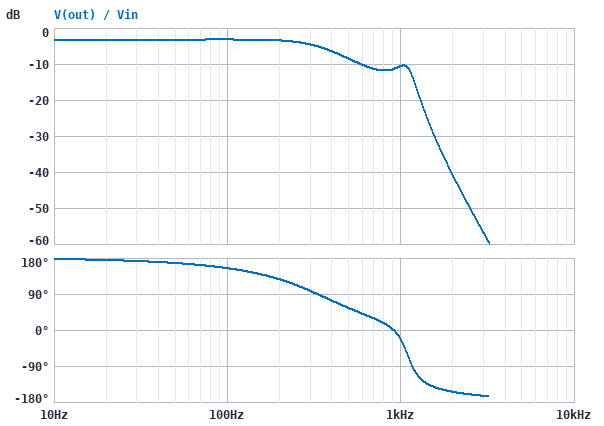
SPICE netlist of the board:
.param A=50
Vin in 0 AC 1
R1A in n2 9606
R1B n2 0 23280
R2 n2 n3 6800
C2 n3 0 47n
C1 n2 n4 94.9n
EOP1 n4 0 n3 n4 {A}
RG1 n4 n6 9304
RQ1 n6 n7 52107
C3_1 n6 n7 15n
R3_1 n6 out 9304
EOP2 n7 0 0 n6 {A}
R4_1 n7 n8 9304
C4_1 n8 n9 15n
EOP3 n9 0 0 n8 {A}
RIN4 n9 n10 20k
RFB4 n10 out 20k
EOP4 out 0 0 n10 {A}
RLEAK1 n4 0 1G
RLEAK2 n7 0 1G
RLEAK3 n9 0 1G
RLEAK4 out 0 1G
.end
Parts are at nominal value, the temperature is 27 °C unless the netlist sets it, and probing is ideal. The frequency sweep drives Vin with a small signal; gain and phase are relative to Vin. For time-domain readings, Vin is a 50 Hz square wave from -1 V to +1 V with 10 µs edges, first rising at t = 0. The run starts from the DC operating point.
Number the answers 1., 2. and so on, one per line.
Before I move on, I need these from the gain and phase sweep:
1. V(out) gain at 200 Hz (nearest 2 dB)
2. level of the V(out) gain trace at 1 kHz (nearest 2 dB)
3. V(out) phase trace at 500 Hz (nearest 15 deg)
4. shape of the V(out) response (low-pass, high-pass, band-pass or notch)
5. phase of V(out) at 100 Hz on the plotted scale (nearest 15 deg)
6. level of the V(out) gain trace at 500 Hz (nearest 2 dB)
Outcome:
1. -4 dB
2. -10 dB
3. 60 deg
4. low-pass
5. 150 deg
6. -8 dB
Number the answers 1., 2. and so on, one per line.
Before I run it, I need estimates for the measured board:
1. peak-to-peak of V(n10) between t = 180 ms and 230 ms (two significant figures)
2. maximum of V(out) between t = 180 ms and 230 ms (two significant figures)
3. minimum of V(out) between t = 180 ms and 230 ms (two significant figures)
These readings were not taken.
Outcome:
1. 31 mV
2. 780 mV
3. -780 mV
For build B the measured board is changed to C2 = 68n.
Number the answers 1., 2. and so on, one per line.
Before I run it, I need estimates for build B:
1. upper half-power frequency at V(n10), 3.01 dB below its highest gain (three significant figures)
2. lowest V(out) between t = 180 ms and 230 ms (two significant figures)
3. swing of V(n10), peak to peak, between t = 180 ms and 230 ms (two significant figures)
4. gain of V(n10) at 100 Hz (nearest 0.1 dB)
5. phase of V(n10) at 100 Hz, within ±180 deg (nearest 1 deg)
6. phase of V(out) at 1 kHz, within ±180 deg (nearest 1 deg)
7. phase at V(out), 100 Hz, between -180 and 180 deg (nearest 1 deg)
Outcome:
1. 248 Hz
2. -700 mV
3. 28 mV
4. -37.6 dB
5. -35 deg
6. -24 deg
7. 145 deg
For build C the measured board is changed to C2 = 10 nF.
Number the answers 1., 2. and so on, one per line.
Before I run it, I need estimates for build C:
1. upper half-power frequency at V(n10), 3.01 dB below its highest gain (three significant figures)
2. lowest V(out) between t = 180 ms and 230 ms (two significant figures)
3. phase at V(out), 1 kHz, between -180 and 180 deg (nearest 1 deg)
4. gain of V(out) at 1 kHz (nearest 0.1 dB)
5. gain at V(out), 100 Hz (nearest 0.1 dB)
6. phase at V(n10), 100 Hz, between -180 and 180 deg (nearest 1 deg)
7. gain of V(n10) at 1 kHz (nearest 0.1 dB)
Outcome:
1. 1.15 kHz
2. -1.8 V
3. -1 deg
4. 6.3 dB
5. -3.0 dB
6. -7 deg
7. -27.7 dB
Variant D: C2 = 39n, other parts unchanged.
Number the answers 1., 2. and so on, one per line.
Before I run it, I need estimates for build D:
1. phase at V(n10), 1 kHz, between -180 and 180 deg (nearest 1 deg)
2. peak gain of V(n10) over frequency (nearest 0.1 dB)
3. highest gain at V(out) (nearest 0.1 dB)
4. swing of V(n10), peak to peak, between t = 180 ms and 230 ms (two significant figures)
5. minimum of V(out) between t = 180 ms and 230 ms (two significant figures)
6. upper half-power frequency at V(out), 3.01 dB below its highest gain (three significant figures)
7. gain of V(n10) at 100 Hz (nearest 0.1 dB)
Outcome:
1. 158 deg
2. -36.9 dB
3. -2.9 dB
4. 33 mV
5. -830 mV
6. 465 Hz
7. -37.1 dB
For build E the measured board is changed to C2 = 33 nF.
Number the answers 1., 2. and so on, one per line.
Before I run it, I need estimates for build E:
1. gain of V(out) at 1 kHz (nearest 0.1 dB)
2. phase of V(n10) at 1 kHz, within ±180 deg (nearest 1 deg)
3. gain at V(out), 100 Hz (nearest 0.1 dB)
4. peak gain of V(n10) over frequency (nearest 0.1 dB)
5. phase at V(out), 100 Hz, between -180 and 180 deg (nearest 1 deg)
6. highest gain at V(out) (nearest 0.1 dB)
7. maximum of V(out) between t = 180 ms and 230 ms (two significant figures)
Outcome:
1. -7.1 dB
2. 159 deg
3. -3.0 dB
4. -36.5 dB
5. 162 deg
6. -2.5 dB
7. 850 mV
